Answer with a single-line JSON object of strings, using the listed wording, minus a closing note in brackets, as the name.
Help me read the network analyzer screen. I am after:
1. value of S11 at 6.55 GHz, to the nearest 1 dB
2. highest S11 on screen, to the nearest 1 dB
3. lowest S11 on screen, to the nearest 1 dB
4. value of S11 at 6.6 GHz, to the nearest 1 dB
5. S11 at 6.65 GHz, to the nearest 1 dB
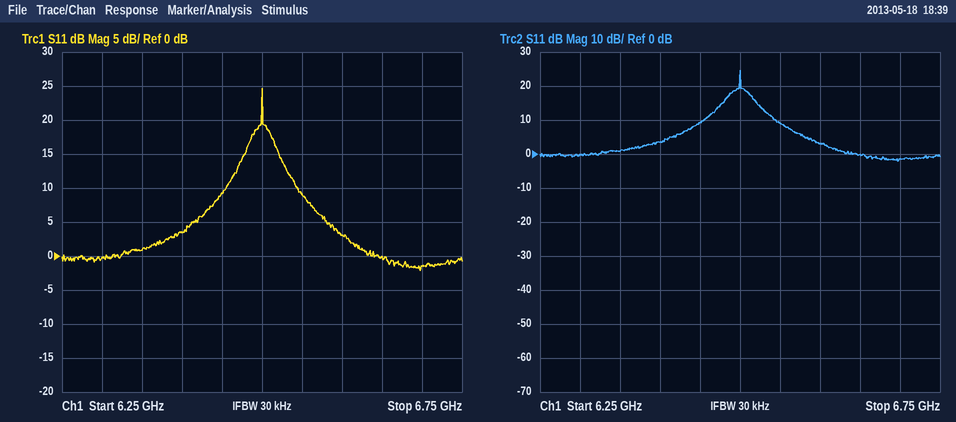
{"value of S11 at 6.55 GHz, to the nearest 1 dB": "9 dB", "highest S11 on screen, to the nearest 1 dB": "25 dB", "lowest S11 on screen, to the nearest 1 dB": "-2 dB", "value of S11 at 6.6 GHz, to the nearest 1 dB": "3 dB", "S11 at 6.65 GHz, to the nearest 1 dB": "0 dB"}
